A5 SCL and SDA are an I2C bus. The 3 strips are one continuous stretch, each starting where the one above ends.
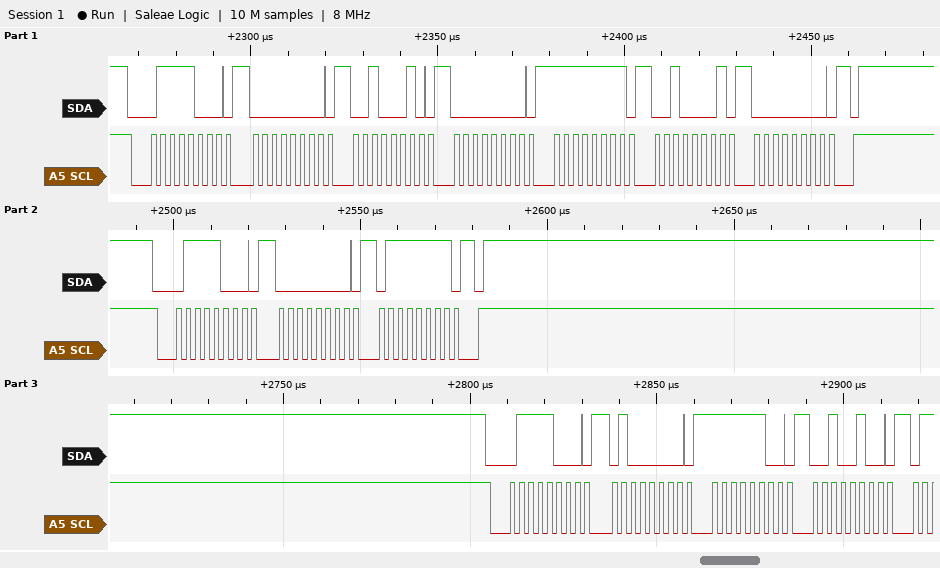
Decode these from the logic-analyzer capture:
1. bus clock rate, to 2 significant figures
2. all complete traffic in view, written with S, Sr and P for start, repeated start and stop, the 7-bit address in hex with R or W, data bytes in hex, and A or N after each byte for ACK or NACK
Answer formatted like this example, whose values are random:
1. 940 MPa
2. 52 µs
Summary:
1. 400 kHz
2. S 3CW A 00 A 22 A 00 A FF A 21 A 00 A P S 3CW A 00 A 7F A P S 3CW A 40 A FC A 24 A
